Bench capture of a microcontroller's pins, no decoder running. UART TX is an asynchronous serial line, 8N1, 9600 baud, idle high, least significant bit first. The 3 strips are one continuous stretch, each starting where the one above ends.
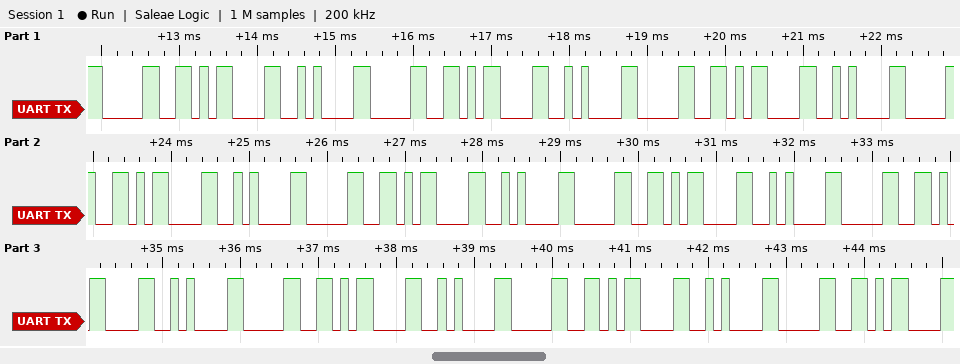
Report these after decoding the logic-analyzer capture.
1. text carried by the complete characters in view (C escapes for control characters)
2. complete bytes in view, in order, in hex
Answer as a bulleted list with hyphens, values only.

- "0\r\n0\r\n0\r\n0\r\n0\r\n0\r\n0\r\n0\r\n0\r\n0\r"
- 0x30 0x0D 0x0A 0x30 0x0D 0x0A 0x30 0x0D 0x0A 0x30 0x0D 0x0A 0x30 0x0D 0x0A 0x30 0x0D 0x0A 0x30 0x0D 0x0A 0x30 0x0D 0x0A 0x30 0x0D 0x0A 0x30 0x0D
